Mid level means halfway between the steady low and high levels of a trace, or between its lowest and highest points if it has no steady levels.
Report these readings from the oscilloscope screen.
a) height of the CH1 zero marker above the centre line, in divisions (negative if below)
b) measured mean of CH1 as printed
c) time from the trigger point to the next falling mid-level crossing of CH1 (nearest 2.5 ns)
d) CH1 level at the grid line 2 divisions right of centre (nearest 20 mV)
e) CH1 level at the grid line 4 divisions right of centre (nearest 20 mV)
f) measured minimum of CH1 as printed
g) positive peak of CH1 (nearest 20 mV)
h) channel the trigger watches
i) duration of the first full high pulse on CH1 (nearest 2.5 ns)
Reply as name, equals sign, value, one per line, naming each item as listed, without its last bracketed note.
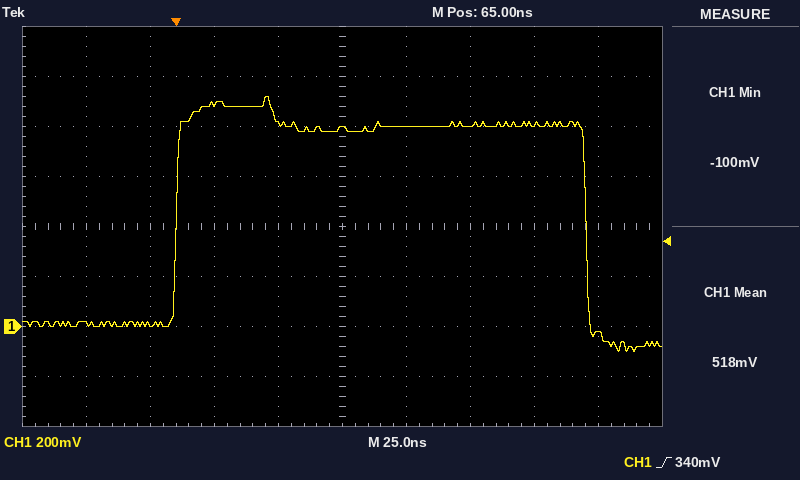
height of the CH1 zero marker above the centre line, in divisions = -2.0 div
measured mean of CH1 as printed = 518 mV
time from the trigger point to the next falling mid-level crossing of CH1 = 160.0 ns
CH1 level at the grid line 2 divisions right of centre = 800 mV
CH1 level at the grid line 4 divisions right of centre = -20 mV
measured minimum of CH1 as printed = -100 mV
positive peak of CH1 = 920 mV
channel the trigger watches = CH1
duration of the first full high pulse on CH1 = 160.0 ns
